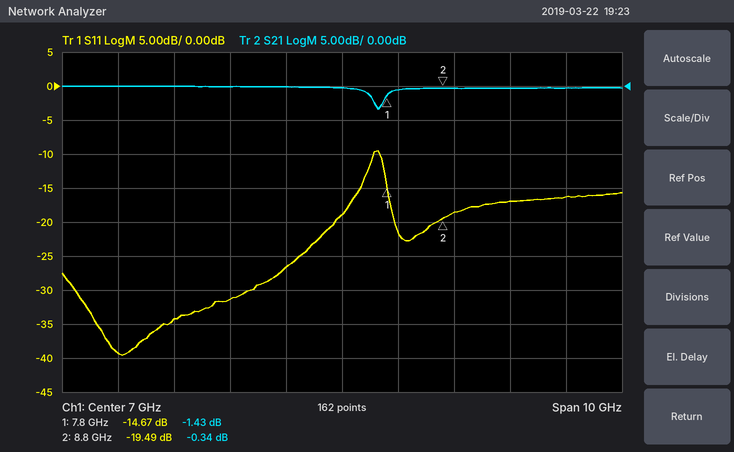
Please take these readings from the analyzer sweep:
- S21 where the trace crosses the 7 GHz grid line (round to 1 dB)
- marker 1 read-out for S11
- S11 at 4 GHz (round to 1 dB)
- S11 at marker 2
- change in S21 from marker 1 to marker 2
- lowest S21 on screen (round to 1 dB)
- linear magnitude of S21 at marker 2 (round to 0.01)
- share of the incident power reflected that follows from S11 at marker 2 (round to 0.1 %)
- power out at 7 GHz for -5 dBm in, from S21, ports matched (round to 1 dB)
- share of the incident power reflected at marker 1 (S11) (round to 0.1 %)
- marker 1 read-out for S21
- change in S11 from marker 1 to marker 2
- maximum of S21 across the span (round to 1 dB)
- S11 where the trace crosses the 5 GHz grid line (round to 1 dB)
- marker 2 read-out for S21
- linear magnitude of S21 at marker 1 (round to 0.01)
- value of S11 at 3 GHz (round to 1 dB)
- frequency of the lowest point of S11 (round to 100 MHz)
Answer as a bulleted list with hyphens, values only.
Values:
- 0 dB
- -14.67 dB
- -34 dB
- -19.49 dB
- 1.09 dB
- -3 dB
- 0.96
- 1.1 %
- -5 dBm
- 3.4 %
- -1.43 dB
- -4.82 dB
- 0 dB
- -31 dB
- -0.34 dB
- 0.85
- -39 dB
- 3.1 GHz
